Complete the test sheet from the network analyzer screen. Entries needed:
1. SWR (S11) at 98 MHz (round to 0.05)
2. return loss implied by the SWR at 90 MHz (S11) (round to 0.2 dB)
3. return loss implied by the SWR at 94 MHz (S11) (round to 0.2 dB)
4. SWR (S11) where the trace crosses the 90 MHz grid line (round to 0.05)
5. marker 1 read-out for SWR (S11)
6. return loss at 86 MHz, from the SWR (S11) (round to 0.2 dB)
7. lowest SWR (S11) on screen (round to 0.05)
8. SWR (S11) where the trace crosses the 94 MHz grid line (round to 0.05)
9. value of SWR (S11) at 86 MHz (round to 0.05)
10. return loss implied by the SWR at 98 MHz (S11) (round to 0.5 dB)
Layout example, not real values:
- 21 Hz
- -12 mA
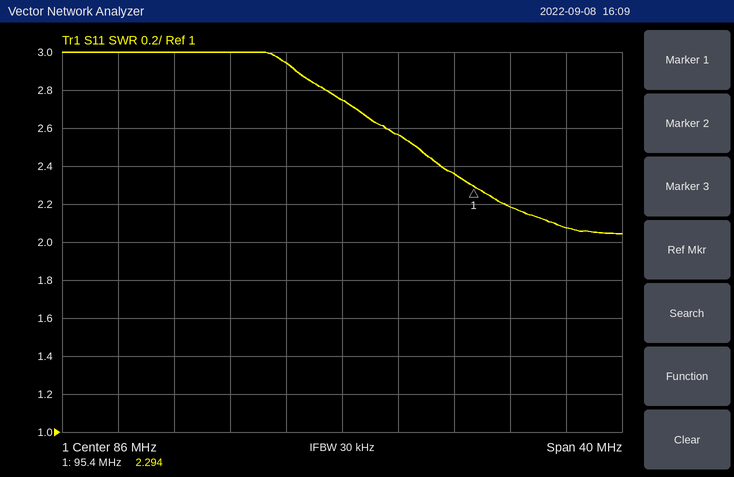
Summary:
- 2.20
- 7.2 dB
- 7.8 dB
- 2.55
- 2.294
- 6.6 dB
- 2.05
- 2.35
- 2.75
- 8.5 dB
